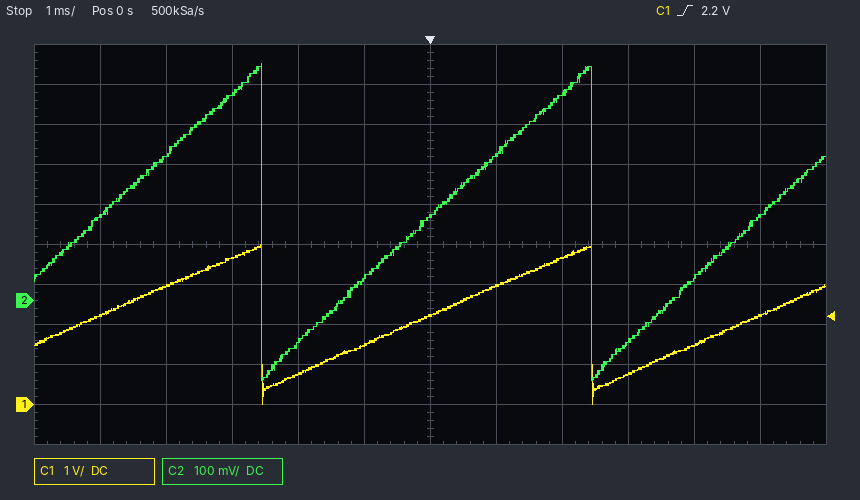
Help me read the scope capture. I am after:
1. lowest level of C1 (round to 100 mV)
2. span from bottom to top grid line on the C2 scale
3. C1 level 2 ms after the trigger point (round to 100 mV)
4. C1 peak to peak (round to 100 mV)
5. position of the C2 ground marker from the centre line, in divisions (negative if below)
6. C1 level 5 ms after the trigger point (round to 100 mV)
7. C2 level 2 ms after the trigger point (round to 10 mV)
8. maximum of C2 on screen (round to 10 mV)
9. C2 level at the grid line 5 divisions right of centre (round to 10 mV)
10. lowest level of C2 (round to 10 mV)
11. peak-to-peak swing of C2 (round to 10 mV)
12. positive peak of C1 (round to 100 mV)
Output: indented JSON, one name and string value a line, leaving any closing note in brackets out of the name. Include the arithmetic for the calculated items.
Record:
{
  "lowest level of C1": "0.0 V",
  "span from bottom to top grid line on the C2 scale": "1 V",
  "C1 level 2 ms after the trigger point": "3.7 V",
  "C1 peak to peak": "4.0 V − (0.0 V) = 4.0 V",
  "position of the C2 ground marker from the centre line, in divisions": "-1.4 div",
  "C1 level 5 ms after the trigger point": "2.2 V",
  "C2 level 2 ms after the trigger point": "520 mV",
  "maximum of C2 on screen": "590 mV",
  "C2 level at the grid line 5 divisions right of centre": "210 mV",
  "lowest level of C2": "-200 mV",
  "peak-to-peak swing of C2": "590 mV − (-200 mV) = 790 mV",
  "positive peak of C1": "4.0 V"
}
